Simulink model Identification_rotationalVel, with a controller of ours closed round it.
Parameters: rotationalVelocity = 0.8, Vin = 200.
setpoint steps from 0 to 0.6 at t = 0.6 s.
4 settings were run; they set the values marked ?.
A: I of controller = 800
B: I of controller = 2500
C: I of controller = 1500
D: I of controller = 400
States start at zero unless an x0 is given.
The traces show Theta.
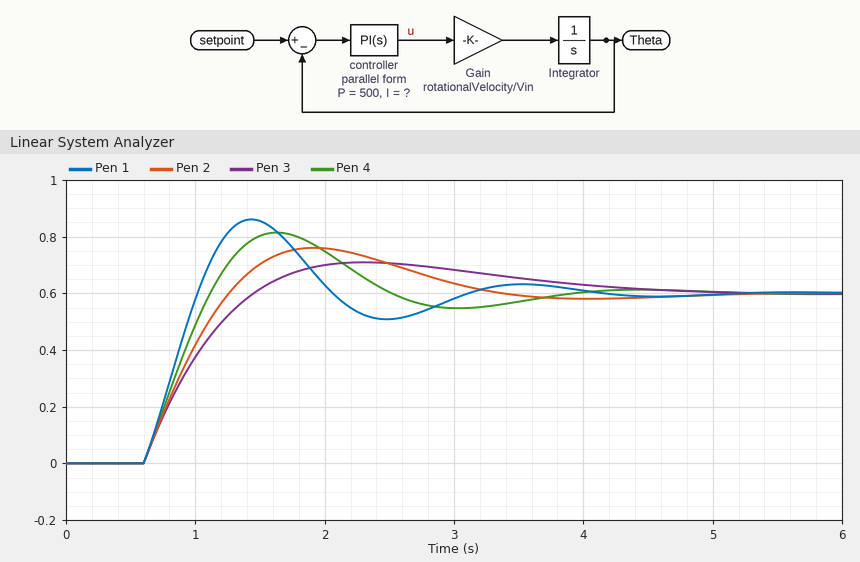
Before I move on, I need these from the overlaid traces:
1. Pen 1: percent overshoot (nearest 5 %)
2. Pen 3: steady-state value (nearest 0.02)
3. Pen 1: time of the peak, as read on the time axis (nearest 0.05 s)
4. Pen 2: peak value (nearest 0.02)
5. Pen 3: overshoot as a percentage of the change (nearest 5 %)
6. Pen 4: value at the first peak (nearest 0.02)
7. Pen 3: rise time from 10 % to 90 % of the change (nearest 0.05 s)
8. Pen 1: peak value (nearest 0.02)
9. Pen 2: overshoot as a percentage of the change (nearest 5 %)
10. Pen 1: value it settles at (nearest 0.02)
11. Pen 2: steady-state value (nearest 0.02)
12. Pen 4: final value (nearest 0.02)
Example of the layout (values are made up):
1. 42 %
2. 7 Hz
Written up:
1. 45 %
2. 0.60
3. 1.45 s
4. 0.76
5. 20 %
6. 0.82
7. 0.65 s
8. 0.86
9. 25 %
10. 0.60
11. 0.60
12. 0.60
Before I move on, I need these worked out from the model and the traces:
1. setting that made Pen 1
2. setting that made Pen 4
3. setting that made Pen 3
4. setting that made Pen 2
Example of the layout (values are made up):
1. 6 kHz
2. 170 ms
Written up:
1. B
2. C
3. D
4. A
